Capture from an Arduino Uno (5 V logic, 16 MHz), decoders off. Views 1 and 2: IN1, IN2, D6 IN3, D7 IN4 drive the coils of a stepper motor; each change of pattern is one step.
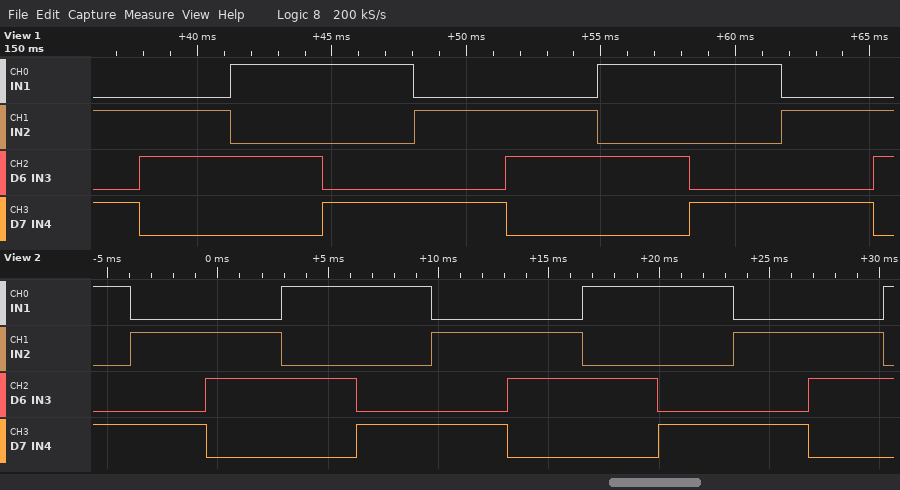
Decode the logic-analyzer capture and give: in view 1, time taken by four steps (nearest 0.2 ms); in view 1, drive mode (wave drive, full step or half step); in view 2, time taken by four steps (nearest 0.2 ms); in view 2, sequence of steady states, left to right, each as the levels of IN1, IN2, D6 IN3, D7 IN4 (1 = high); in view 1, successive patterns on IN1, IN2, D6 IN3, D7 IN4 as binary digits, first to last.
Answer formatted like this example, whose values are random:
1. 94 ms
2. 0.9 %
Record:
1. 13.6 ms
2. full step
3. 13.6 ms
4. 1001 0101 0110 1010 1001 0101 0110 1010 1001 0101 0110 1010
5. 0101 0110 1010 1001 0101 0110 1010 1001 0101 0110
